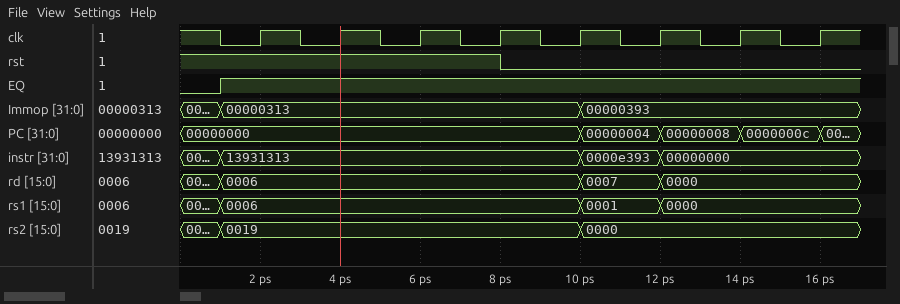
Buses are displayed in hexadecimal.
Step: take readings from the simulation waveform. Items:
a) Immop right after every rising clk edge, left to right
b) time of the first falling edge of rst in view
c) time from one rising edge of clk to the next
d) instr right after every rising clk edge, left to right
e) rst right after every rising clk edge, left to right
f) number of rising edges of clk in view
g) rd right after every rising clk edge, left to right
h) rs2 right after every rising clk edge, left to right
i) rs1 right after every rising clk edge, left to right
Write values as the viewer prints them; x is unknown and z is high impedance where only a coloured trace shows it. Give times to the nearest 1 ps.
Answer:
00000313, 00000313, 00000313, 00000313, 00000393, 00000393, 00000393, 00000393
8 ps
2 ps
13931313, 13931313, 13931313, 13931313, 0000e393, 00000000, 00000000, 00000000
1 1 1 0 0 0 0 0
8
0006, 0006, 0006, 0006, 0007, 0000, 0000, 0000
0019, 0019, 0019, 0019, 0000, 0000, 0000, 0000
0006, 0006, 0006, 0006, 0001, 0000, 0000, 0000
